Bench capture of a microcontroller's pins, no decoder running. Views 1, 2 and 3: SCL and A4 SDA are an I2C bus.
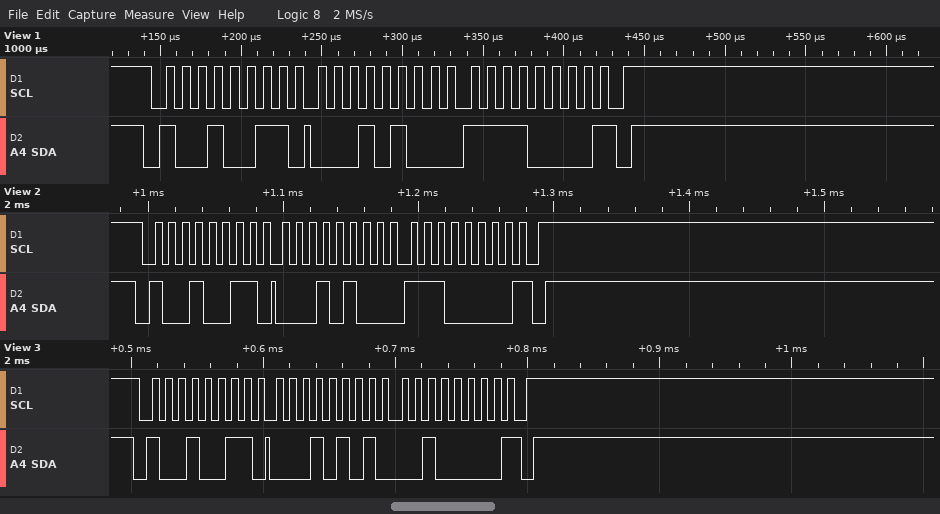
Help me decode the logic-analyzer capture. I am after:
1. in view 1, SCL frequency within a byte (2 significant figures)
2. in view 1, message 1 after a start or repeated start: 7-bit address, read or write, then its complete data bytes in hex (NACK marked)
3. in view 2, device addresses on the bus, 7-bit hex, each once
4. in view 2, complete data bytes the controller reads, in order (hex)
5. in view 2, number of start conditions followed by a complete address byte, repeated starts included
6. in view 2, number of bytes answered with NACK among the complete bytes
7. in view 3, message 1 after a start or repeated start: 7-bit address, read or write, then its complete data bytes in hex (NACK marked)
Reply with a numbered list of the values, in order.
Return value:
1. 100 kHz
2. 0x49 read: 14 F0 NACK
3. 0x49
4. 14 E0
5. 1
6. 1
7. 0x49 read: 15 20 NACK
